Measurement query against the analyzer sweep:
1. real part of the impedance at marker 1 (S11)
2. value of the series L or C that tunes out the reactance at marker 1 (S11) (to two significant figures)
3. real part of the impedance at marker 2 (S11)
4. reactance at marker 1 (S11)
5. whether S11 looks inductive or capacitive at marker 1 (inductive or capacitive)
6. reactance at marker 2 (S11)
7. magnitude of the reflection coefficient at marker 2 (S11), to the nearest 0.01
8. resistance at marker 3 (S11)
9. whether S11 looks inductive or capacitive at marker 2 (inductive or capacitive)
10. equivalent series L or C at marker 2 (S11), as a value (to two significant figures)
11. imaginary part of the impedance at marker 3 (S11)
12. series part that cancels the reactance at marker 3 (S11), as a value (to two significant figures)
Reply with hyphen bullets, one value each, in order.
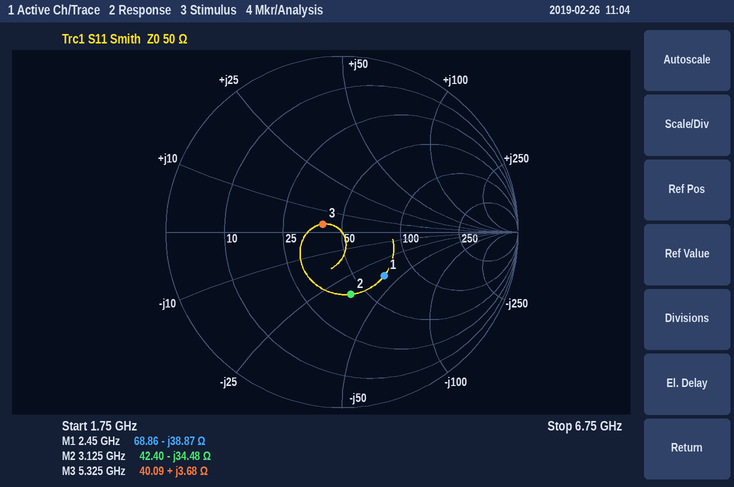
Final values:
- 68.86 Ω
- 2.5 nH
- 42.40 Ω
- -38.87 Ω
- capacitive
- -34.48 Ω
- 0.36
- 40.09 Ω
- capacitive
- 1.5 pF
- +3.68 Ω
- 8.1 pF
